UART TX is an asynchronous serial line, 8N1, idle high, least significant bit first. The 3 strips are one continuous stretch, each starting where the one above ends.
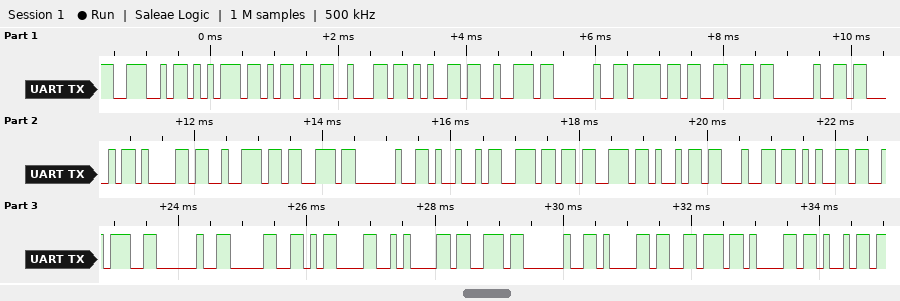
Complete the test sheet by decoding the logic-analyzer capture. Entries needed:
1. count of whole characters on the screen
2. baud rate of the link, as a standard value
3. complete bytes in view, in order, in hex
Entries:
32
9600 baud
0x4E 0x75 0x6D 0x62 0x65 0x72 0x20 0x6F 0x66 0x20 0x43 0x61 0x72 0x73 0x20 0x49 0x6E 0x73 0x69 0x64 0x65 0x3A 0x20 0x30 0x0D 0x0A 0x73 0x20 0x61 0x76 0x61 0x69
